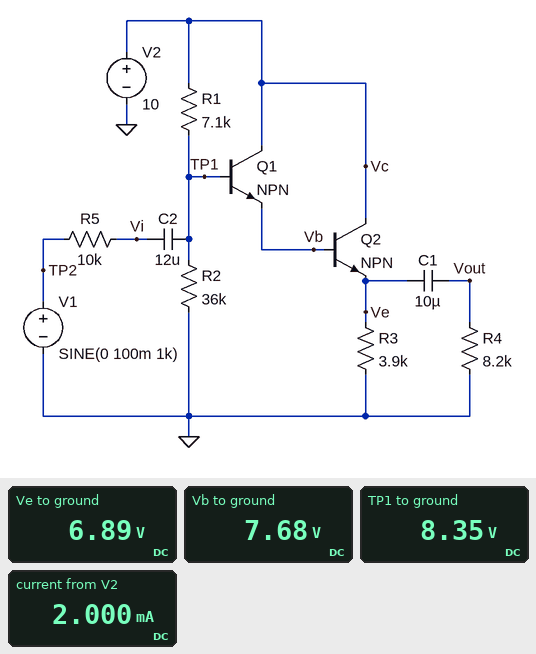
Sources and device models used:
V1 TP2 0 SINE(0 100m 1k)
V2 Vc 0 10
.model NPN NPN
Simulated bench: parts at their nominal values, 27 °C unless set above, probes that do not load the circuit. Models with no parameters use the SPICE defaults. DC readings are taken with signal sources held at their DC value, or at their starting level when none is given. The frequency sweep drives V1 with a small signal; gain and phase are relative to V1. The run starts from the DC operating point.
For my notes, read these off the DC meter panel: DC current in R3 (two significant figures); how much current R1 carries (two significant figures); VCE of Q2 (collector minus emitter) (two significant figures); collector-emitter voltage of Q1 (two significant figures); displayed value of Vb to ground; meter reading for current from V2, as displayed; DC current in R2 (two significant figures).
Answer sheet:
1.8 mA
230 µA
3.1 V
2.3 V
7.68 V
2.000 mA
230 µA
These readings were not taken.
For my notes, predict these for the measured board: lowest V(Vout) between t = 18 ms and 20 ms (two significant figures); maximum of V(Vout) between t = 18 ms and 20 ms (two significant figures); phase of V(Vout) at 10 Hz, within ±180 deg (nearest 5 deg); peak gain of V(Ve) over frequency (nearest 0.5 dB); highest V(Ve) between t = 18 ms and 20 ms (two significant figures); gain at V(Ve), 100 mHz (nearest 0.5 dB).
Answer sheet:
-37 mV
37 mV
15 deg
-8.5 dB
6.9 V
-27.0 dB
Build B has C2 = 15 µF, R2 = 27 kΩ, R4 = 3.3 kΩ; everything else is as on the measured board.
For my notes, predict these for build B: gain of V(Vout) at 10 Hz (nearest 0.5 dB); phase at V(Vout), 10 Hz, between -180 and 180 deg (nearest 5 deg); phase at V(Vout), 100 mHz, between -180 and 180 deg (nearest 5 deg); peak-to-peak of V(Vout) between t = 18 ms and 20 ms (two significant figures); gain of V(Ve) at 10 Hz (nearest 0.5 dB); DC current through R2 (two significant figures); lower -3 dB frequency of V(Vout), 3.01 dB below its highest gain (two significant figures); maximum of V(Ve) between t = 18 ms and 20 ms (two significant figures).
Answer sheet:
-10.0 dB
30 deg
170 deg
71 mV
-9.0 dB
290 µA
4.9 Hz
6.5 V
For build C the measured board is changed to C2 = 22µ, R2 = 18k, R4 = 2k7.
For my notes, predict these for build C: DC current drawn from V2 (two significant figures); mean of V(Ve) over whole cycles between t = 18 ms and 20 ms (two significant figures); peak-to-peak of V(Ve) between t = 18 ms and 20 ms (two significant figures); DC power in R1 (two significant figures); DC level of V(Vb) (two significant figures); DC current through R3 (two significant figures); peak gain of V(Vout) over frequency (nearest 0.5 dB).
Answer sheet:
1.9 mA
5.7 V
66 mV
1.1 mW
6.5 V
1.5 mA
-9.5 dB
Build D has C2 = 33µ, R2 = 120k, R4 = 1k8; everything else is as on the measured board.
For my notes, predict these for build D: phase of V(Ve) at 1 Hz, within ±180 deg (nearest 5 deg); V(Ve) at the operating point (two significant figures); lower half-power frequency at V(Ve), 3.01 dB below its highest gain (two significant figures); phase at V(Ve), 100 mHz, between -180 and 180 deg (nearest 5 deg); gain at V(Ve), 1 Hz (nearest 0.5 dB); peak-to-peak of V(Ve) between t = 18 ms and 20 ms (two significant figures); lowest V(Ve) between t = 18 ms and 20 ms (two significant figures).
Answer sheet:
15 deg
8.0 V
290 mHz
70 deg
-8.5 dB
79 mV
7.9 V
